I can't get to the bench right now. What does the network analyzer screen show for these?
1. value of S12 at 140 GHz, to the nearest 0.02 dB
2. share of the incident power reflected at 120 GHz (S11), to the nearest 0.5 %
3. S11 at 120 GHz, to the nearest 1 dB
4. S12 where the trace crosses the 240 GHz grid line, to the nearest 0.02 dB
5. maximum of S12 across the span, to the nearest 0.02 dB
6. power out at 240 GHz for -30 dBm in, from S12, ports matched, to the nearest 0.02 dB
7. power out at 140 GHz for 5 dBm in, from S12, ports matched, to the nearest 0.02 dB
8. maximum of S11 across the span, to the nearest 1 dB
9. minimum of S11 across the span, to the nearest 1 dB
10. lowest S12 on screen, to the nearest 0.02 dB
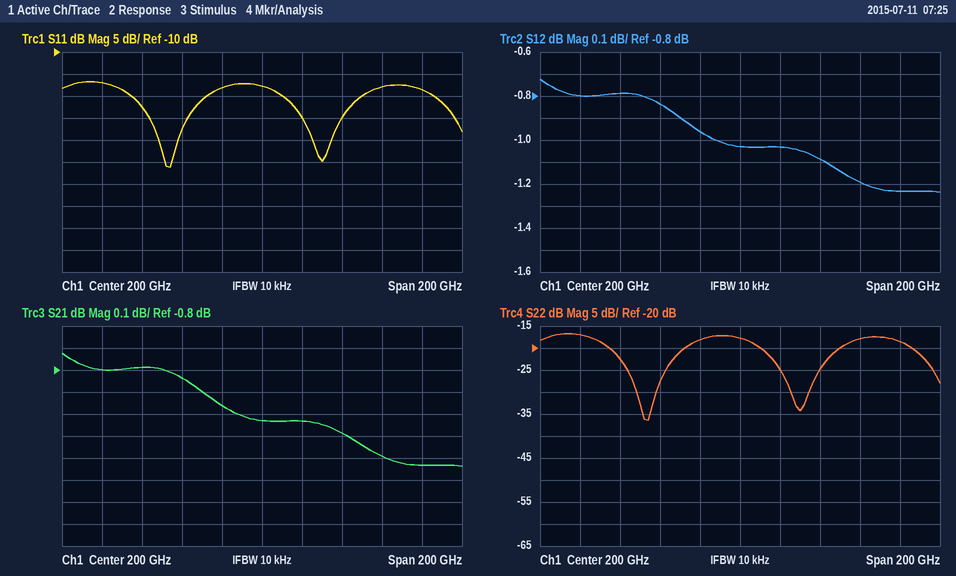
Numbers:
-0.78 dB
2.0 %
-17 dB
-1.08 dB
-0.72 dB
-31.08 dBm
4.22 dBm
-17 dB
-36 dB
-1.24 dB
